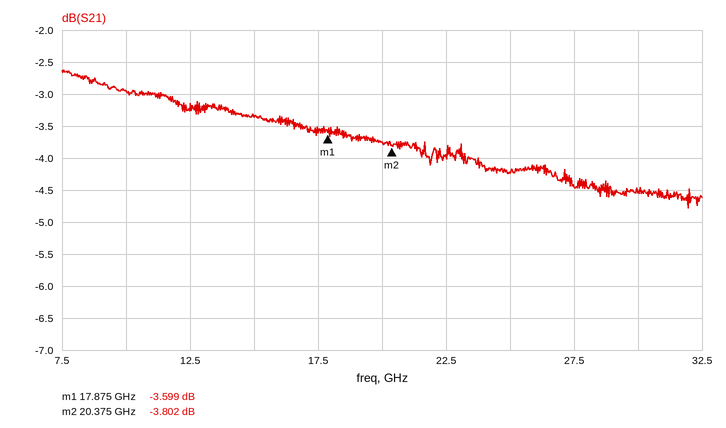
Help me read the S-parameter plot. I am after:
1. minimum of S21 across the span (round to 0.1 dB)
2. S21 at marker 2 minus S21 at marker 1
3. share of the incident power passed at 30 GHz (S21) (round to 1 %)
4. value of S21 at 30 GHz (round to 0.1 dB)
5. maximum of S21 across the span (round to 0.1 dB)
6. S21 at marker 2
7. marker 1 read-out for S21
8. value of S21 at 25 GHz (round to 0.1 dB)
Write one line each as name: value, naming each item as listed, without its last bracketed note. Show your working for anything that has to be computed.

minimum of S21 across the span: -4.8 dB
S21 at marker 2 minus S21 at marker 1: -3.802 − (-3.599) = -0.203 dB
share of the incident power passed at 30 GHz (S21): 10^(-4.5/10) ≈ 35 %
value of S21 at 30 GHz: -4.5 dB
maximum of S21 across the span: -2.6 dB
S21 at marker 2: -3.802 dB
marker 1 read-out for S21: -3.599 dB
value of S21 at 25 GHz: -4.2 dB
